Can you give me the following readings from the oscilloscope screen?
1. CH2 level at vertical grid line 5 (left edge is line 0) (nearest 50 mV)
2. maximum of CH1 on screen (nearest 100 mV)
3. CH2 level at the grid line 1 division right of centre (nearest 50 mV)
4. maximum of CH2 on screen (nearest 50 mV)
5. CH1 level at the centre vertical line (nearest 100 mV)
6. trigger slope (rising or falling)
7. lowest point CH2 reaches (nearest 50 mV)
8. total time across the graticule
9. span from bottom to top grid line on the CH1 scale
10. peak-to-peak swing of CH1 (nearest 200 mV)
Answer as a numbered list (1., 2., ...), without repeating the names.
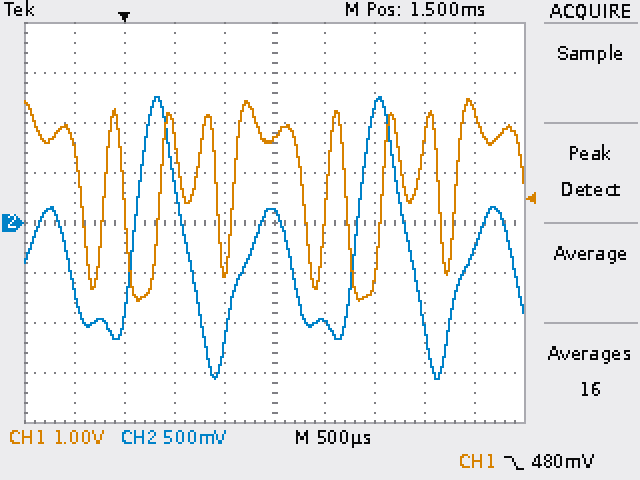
1. 100 mV
2. 2.5 V
3. -1.00 V
4. 1.25 V
5. 1.7 V
6. falling
7. -1.55 V
8. 5 ms
9. 8 V
10. 4.0 V
